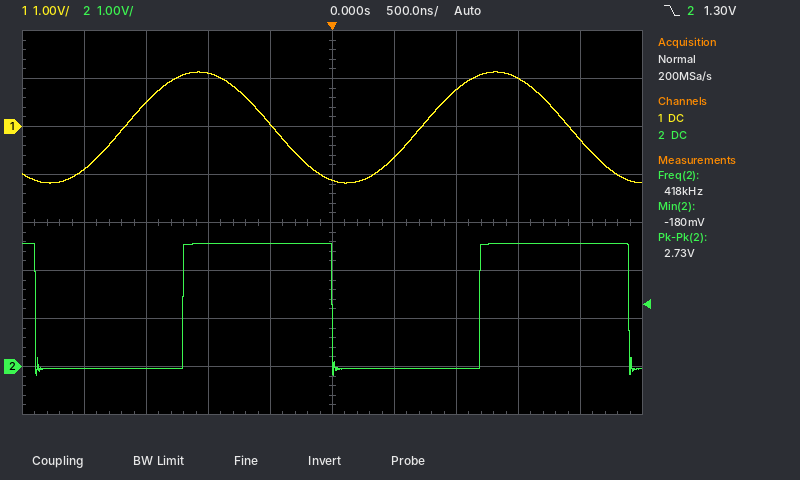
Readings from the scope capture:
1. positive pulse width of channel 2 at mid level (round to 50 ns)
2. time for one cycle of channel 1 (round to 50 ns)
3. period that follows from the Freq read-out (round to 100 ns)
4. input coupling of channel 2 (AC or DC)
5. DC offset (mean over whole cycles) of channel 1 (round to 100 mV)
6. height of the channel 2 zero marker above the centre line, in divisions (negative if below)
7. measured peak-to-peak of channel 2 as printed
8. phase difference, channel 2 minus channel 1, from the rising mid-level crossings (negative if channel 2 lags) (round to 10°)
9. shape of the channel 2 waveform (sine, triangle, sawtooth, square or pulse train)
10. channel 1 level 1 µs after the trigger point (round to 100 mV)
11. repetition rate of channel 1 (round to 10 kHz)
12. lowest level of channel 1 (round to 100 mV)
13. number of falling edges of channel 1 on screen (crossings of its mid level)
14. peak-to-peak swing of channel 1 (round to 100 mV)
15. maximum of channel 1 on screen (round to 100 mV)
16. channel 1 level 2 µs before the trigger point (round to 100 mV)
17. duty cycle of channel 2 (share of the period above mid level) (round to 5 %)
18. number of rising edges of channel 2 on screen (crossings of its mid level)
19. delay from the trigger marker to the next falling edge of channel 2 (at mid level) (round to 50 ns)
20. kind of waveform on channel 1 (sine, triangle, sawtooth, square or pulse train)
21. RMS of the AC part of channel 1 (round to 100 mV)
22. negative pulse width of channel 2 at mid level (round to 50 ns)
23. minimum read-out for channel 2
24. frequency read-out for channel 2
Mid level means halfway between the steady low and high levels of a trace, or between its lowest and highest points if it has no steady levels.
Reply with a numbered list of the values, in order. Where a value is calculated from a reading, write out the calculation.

1. 1.20 µs
2. 2.40 µs
3. 1 / 418 kHz ≈ 2.4 µs
4. DC
5. (1.1 V + (-1.2 V)) / 2 ≈ 0.0 V
6. -3.0 div
7. 2.73 V
8. -70°
9. square
10. 800 mV
11. 1 / 2.40 µs ≈ 417 kHz, so 420 kHz to the nearest 10 kHz
12. -1.2 V
13. 2
14. 1.1 V − (-1.2 V) = 2.3 V
15. 1.1 V
16. -900 mV
17. 50 %
18. 2
19. 2.40 µs
20. sine
21. 2.3 V / (2√2) ≈ 813 mV, so 800 mV to the nearest 100 mV
22. 1.20 µs
23. -180 mV
24. 418 kHz
